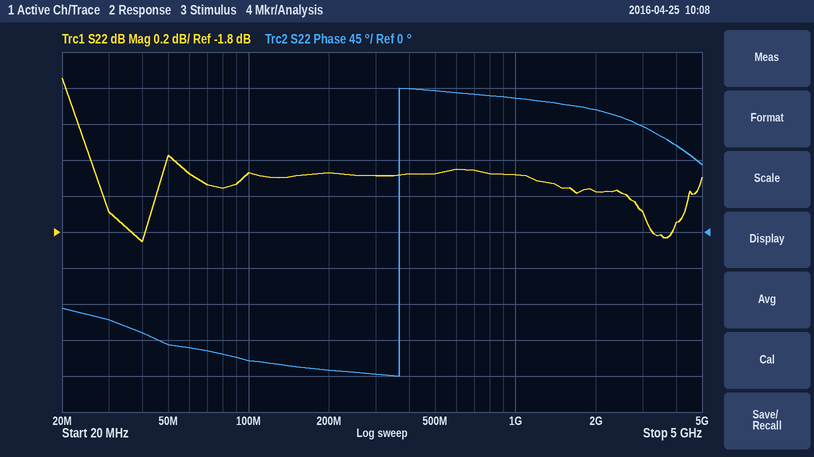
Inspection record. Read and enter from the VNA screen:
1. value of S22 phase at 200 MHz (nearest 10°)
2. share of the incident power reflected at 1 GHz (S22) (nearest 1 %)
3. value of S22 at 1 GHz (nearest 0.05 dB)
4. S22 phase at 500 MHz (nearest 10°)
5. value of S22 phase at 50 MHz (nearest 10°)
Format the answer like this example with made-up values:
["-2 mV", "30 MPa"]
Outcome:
["-170°", "71 %", "-1.50 dB", "180°", "-140°"]
